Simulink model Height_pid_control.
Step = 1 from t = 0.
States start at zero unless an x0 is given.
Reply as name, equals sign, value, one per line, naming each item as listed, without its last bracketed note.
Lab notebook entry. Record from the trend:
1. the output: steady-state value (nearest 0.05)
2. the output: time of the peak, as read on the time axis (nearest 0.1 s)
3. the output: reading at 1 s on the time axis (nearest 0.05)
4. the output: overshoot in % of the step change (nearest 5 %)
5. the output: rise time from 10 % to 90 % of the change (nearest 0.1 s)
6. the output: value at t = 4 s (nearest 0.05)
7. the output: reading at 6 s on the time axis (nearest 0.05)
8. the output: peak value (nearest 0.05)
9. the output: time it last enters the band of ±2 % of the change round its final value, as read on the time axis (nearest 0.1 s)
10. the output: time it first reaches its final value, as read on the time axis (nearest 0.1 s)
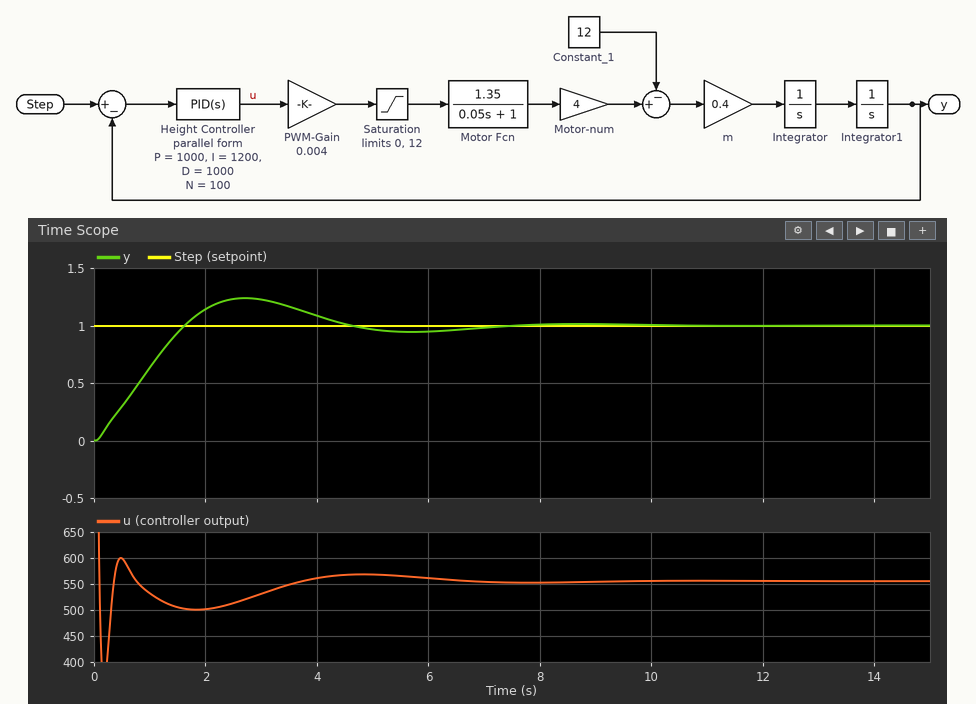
the output: steady-state value = 1.00
the output: time of the peak, as read on the time axis = 2.7 s
the output: reading at 1 s on the time axis = 0.65
the output: overshoot in % of the step change = 25 %
the output: rise time from 10 % to 90 % of the change = 1.2 s
the output: value at t = 4 s = 1.10
the output: reading at 6 s on the time axis = 0.95
the output: peak value = 1.25
the output: time it last enters the band of ±2 % of the change round its final value, as read on the time axis = 7.0 s
the output: time it first reaches its final value, as read on the time axis = 1.6 s
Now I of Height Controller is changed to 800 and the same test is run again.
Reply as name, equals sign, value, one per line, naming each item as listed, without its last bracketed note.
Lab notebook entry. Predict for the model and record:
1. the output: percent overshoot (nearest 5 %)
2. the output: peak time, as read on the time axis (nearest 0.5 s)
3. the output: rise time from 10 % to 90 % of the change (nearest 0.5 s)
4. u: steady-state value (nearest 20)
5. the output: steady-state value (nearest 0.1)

the output: percent overshoot = 15 %
the output: peak time, as read on the time axis = 3.5 s
the output: rise time from 10 % to 90 % of the change = 1.5 s
u: steady-state value = 560
the output: steady-state value = 1.0
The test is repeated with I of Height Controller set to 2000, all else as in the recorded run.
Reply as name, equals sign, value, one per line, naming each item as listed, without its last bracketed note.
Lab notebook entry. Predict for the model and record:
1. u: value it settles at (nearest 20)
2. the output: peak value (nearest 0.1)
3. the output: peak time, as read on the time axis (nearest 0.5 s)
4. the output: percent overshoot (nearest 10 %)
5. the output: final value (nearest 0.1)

u: value it settles at = 560
the output: peak value = 1.4
the output: peak time, as read on the time axis = 2.0 s
the output: percent overshoot = 40 %
the output: final value = 1.0
